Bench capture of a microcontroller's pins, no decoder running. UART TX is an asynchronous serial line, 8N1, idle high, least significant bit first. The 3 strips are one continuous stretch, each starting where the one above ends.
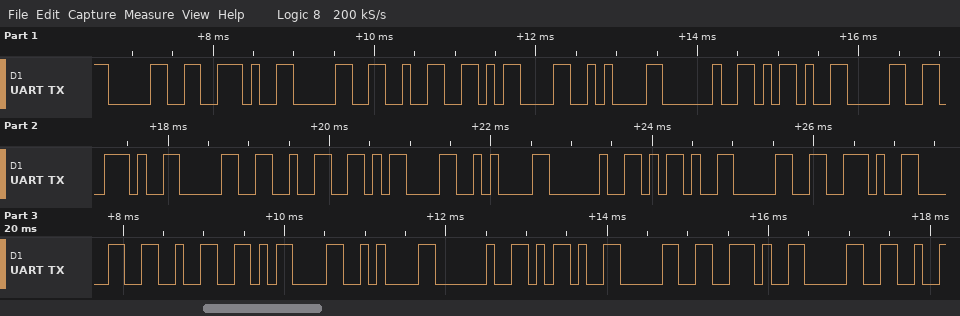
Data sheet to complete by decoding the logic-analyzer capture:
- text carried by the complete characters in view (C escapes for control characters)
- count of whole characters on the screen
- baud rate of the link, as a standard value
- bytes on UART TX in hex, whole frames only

"0.02\r\n -0.02\r\n -0.02\r\n -0.0"
27
9600 baud
0x30 0x2E 0x30 0x32 0x0D 0x0A 0x20 0x2D 0x30 0x2E 0x30 0x32 0x0D 0x0A 0x20 0x2D 0x30 0x2E 0x30 0x32 0x0D 0x0A 0x20 0x2D 0x30 0x2E 0x30
